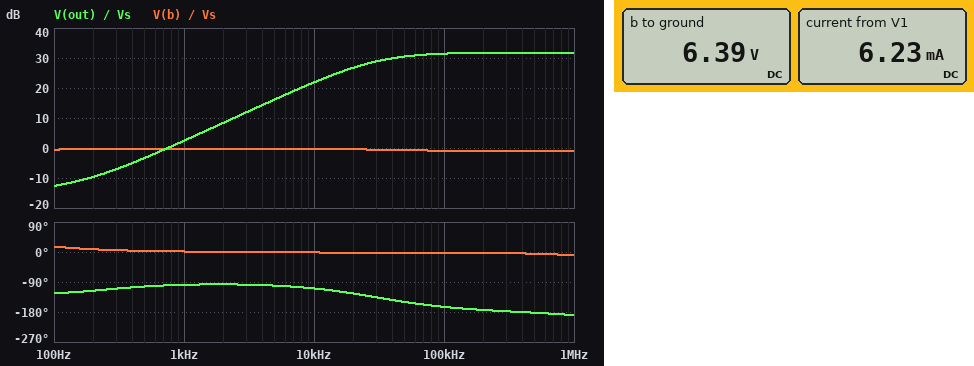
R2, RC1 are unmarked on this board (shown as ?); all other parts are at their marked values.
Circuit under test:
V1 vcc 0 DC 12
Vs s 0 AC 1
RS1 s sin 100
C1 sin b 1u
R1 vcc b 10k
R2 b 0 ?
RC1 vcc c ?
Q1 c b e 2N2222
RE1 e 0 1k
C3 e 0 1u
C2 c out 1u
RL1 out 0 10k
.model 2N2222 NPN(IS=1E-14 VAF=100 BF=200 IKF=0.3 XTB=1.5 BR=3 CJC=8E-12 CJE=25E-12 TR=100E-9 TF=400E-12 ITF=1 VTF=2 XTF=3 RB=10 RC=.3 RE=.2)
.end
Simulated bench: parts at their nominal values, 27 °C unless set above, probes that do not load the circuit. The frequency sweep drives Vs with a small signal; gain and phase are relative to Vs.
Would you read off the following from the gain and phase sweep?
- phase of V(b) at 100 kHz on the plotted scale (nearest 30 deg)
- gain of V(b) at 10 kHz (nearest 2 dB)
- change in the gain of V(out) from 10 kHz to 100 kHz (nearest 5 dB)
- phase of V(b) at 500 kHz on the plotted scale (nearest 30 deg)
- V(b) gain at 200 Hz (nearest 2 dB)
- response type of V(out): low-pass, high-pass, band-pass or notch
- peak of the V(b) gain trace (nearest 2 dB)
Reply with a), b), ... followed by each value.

a) 0 deg
b) 0 dB
c) 10 dB
d) 0 deg
e) 0 dB
f) high-pass
g) 0 dB
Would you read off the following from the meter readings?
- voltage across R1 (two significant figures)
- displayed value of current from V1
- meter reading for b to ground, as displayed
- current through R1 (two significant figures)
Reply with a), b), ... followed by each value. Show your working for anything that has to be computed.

a) 12 V - 6.39 V = 5.6 V
b) 6.23 mA
c) 6.39 V
d) (12 V - 6.39 V) / 10 kΩ = 560 µA
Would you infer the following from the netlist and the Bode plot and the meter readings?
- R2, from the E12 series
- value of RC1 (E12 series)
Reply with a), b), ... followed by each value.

a) 12 kΩ
b) 220 Ω
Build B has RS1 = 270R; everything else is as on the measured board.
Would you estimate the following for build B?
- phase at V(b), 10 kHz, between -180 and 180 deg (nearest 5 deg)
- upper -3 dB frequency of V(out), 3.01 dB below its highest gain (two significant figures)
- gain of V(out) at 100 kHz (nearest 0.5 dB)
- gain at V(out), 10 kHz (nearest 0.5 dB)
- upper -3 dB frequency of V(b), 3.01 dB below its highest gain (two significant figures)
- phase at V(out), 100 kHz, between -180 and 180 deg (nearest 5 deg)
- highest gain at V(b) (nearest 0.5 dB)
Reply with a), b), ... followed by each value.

a) -5 deg
b) 2.4 MHz
c) 30.0 dB
d) 21.5 dB
e) 1.3 MHz
f) -170 deg
g) -0.5 dB
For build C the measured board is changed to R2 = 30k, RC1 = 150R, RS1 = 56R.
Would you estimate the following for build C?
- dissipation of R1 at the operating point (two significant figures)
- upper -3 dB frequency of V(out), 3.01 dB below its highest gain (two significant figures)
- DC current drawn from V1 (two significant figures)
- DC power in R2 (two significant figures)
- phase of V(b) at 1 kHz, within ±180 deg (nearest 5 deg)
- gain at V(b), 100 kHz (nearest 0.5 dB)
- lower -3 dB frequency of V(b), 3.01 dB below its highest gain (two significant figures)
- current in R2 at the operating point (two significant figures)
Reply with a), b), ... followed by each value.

a) 1.1 mW
b) 7.1 MHz
c) 8.3 mA
d) 2.5 mW
e) 0 deg
f) -0.5 dB
g) 22 Hz
h) 290 µA
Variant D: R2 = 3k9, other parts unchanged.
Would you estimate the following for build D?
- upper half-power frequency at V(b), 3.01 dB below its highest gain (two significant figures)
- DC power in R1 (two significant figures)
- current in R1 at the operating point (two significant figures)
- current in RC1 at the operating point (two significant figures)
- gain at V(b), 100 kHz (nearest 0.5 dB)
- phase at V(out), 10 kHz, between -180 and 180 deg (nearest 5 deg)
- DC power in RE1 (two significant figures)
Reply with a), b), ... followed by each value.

a) 9.1 MHz
b) 7.5 mW
c) 870 µA
d) 2.6 mA
e) -0.5 dB
f) -125 deg
g) 7.0 mW
